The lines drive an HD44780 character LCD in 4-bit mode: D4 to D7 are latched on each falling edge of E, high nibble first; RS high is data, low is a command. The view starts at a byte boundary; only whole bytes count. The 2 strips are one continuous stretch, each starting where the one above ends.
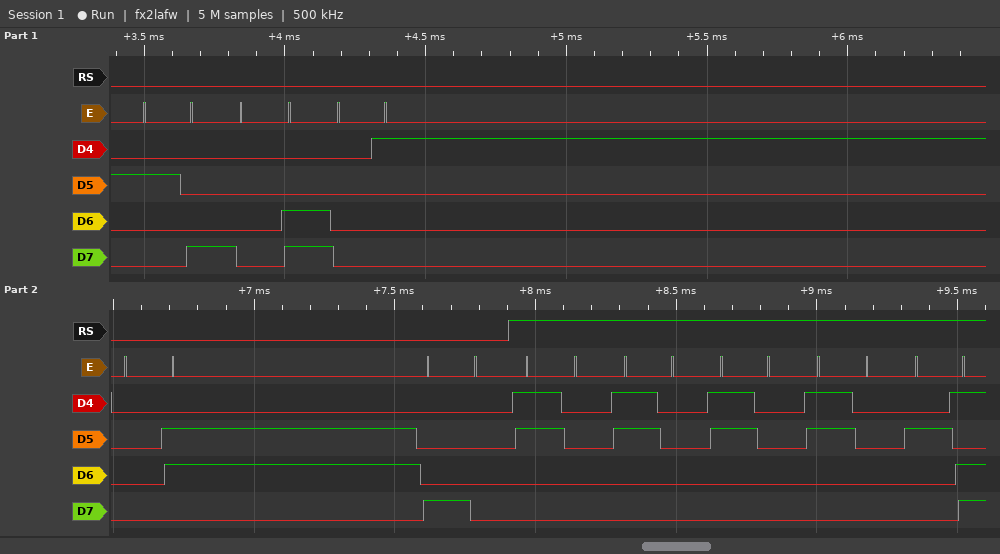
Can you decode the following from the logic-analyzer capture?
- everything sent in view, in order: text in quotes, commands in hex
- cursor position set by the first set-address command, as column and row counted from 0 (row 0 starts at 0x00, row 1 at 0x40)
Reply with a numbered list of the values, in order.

1. 0x28 0x0C 0x01 0x06 0x80 "0000-"
2. column 0, row 0
